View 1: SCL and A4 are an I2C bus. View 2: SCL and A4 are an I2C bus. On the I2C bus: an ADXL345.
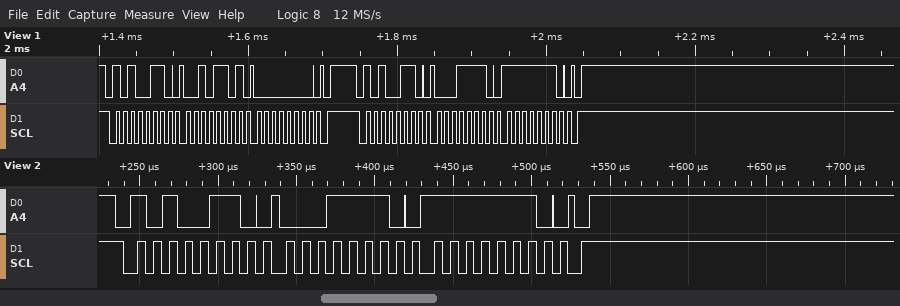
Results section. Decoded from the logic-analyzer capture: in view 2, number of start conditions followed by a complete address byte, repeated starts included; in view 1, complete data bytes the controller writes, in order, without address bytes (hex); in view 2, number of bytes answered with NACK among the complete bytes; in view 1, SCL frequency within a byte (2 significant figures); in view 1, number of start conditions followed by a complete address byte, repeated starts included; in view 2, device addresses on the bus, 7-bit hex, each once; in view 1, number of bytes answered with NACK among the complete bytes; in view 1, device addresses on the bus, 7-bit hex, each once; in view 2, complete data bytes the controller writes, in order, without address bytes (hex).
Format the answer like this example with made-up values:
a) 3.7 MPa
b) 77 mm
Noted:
a) 1
b) 2D 00 1E FE
c) 0
d) 100 kHz
e) 2
f) 0x53
g) 0
h) 0x53
i) 1E FE
